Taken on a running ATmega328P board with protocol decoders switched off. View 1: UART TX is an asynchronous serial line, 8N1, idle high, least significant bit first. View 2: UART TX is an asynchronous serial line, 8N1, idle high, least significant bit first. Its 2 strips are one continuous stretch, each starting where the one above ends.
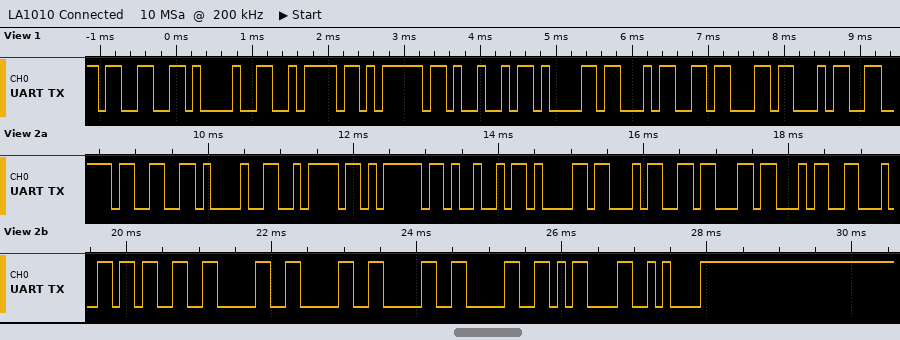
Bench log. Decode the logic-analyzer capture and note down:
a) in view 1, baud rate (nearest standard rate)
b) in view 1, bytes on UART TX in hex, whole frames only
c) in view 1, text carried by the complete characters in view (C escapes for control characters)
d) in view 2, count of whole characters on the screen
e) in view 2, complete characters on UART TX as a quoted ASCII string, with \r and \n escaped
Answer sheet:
9600 baud
0x33 0x21 0x7A 0x7D 0x49 0x61 0x34 0x63 0x34
"3!z}Ia4c4"
17
"3!z}Ia4c4d30000\r\n"
